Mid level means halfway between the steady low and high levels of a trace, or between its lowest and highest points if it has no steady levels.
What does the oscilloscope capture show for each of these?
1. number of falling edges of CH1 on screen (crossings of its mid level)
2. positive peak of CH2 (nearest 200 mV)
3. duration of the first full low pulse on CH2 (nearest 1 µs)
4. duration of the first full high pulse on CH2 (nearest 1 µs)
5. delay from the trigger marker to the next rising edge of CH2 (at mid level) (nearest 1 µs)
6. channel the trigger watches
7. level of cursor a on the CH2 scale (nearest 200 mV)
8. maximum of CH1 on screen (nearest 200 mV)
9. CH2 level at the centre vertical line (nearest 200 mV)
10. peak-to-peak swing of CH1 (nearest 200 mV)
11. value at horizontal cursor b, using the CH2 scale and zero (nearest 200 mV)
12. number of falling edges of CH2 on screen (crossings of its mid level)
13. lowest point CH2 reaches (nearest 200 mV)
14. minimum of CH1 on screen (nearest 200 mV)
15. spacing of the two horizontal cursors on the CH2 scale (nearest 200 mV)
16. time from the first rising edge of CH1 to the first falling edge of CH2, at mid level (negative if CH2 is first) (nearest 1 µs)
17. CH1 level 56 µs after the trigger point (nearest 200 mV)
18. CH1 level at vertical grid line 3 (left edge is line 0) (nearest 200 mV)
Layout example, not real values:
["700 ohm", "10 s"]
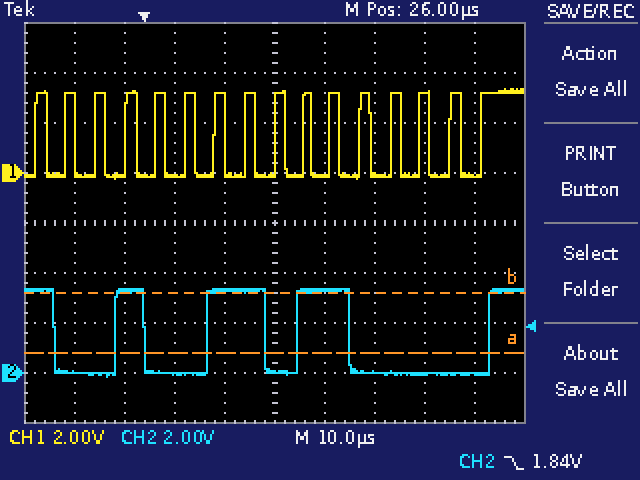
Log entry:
["15", "3.4 V", "12 µs", "6 µs", "13 µs", "CH2", "800 mV", "3.4 V", "0.0 V", "3.6 V", "3.2 V", "4", "-200 mV", "-200 mV", "2.4 V", "+4 µs", "3.2 V", "-200 mV"]
